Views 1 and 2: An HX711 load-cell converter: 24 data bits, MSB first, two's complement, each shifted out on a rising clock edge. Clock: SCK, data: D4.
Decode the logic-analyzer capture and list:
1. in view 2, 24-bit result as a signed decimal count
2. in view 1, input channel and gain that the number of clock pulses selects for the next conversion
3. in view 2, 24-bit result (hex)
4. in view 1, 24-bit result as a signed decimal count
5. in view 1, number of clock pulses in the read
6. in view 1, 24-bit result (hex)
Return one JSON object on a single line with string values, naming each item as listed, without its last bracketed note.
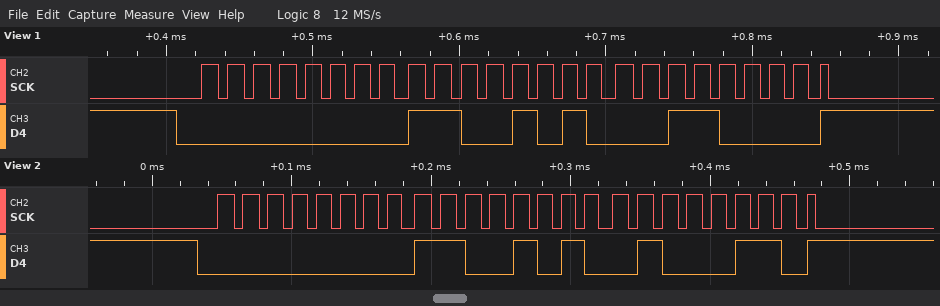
{"in view 2, 24-bit result as a signed decimal count": "51782", "in view 1, input channel and gain that the number of clock pulses selects for the next conversion": "channel A, gain 128", "in view 2, 24-bit result": "0x00CA46", "in view 1, 24-bit result as a signed decimal count": "51760", "in view 1, number of clock pulses in the read": "25", "in view 1, 24-bit result": "0x00CA30"}
